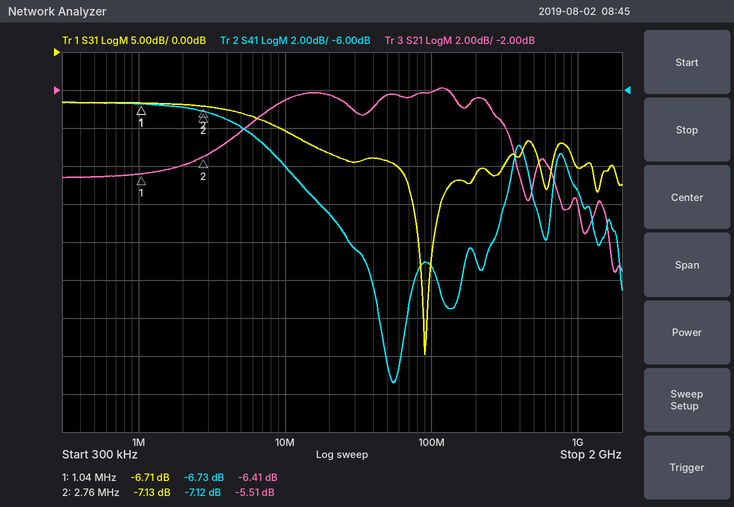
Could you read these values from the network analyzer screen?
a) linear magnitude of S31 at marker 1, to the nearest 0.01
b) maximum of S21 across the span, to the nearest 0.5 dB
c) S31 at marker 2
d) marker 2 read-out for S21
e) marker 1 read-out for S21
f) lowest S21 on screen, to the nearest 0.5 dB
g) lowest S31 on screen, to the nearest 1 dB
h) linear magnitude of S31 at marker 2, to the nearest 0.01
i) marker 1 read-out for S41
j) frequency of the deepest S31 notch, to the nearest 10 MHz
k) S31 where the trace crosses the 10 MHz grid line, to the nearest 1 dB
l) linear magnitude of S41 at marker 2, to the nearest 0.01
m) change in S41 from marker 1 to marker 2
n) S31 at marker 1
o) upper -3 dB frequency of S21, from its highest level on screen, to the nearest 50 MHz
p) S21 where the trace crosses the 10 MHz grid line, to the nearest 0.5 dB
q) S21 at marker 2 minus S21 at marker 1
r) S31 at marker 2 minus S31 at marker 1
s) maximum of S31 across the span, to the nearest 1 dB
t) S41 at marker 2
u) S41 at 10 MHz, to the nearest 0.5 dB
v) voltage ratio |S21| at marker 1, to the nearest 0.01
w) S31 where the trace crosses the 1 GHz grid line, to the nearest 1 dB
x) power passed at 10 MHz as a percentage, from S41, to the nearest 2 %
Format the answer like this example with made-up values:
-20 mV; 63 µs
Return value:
0.46; -2.0 dB; -7.13 dB; -5.51 dB; -6.41 dB; -11.5 dB; -40 dB; 0.44; -6.73 dB; 90 MHz; -10 dB; 0.44; -0.39 dB; -6.71 dB; 350 MHz; -2.5 dB; 0.90 dB; -0.42 dB; -7 dB; -7.12 dB; -10.0 dB; 0.48; -15 dB; 10 %
